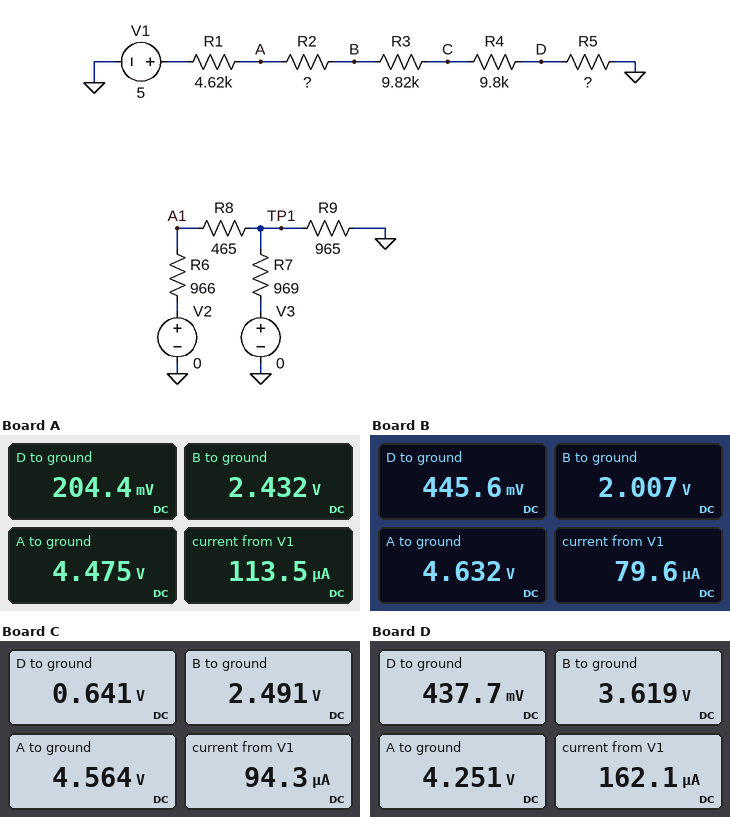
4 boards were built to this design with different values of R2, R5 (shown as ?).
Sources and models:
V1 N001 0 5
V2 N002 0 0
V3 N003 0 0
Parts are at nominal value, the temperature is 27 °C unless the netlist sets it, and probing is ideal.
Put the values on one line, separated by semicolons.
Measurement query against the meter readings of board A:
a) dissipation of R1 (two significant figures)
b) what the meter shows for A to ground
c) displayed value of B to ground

60 µW; 4.475 V; 2.432 V
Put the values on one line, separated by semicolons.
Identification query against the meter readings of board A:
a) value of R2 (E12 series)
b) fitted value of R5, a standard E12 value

18 kΩ; 1.8 kΩ
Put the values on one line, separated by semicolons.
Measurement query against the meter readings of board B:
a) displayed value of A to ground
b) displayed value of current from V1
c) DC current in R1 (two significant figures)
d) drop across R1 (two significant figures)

4.632 V; 79.6 µA; 80 µA; 370 mV
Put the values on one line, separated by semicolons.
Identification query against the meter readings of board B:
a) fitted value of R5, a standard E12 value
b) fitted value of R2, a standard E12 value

5.6 kΩ; 33 kΩ
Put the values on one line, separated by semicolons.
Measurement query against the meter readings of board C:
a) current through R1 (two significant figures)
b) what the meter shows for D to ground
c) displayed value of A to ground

94 µA; 0.641 V; 4.564 V
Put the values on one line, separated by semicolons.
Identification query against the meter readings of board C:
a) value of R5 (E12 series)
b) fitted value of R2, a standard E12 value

6.8 kΩ; 22 kΩ
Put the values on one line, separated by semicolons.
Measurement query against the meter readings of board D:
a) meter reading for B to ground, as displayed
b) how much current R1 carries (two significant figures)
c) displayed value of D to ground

3.619 V; 160 µA; 437.7 mV
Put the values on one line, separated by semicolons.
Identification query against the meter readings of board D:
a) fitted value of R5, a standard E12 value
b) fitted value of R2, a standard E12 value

2.7 kΩ; 3.9 kΩ
